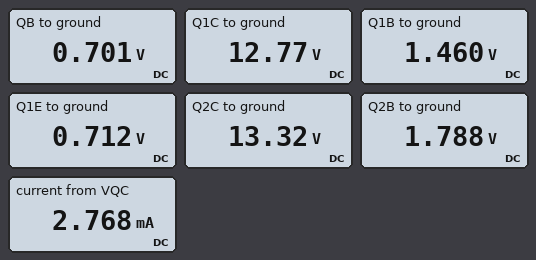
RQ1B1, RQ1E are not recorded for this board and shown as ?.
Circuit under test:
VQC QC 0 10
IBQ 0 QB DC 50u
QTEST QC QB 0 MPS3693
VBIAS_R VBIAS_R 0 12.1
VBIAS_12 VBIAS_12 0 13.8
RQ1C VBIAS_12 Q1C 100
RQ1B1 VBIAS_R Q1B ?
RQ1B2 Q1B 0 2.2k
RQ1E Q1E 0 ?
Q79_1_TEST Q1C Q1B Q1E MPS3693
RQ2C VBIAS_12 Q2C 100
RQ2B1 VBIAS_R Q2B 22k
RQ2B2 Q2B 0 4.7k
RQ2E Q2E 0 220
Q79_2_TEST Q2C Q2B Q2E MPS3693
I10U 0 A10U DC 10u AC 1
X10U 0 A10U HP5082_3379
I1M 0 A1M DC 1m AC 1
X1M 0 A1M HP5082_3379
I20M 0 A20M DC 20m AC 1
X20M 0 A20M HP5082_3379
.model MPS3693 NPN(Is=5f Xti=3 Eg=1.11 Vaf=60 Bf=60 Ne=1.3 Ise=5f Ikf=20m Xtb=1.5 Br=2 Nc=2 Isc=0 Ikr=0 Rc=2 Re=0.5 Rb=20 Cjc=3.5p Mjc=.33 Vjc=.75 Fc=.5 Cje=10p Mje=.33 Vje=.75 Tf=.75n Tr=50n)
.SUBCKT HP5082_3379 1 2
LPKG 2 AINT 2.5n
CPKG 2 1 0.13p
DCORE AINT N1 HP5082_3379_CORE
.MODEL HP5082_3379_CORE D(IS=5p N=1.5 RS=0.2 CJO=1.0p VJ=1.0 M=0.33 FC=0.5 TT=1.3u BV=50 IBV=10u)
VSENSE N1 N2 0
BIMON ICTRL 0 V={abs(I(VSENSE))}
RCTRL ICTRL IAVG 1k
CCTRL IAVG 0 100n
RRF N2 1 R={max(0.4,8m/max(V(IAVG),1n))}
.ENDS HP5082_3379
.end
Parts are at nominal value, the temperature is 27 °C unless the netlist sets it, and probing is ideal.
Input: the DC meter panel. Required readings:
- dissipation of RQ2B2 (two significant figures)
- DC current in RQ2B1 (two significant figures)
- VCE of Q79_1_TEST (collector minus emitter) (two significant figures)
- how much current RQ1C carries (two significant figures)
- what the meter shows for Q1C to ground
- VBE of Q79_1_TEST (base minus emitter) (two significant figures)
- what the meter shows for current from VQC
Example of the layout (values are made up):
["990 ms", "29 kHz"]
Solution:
["680 µW", "470 µA", "12 V", "10 mA", "12.77 V", "750 mV", "2.768 mA"]
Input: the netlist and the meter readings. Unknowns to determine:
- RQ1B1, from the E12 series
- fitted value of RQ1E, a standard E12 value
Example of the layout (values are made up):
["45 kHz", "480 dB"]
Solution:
["12 kΩ", "68 Ω"]
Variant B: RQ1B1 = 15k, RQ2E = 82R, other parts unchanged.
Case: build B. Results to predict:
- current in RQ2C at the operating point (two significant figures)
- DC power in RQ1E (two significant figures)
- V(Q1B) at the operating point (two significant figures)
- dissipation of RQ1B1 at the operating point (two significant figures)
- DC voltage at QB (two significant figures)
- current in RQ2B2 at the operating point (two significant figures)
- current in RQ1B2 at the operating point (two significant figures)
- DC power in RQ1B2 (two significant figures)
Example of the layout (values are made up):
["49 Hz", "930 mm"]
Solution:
["8.5 mA", "4.0 mW", "1.3 V", "7.8 mW", "700 mV", "310 µA", "570 µA", "720 µW"]
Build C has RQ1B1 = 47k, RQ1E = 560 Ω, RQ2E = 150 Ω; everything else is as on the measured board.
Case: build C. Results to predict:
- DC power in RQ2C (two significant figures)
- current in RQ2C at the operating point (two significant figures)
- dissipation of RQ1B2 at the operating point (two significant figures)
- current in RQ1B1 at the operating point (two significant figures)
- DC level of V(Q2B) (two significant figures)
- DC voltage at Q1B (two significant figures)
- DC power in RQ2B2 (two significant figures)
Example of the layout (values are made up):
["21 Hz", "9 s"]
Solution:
["3.8 mW", "6.2 mA", "130 µW", "250 µA", "1.7 V", "540 mV", "590 µW"]
